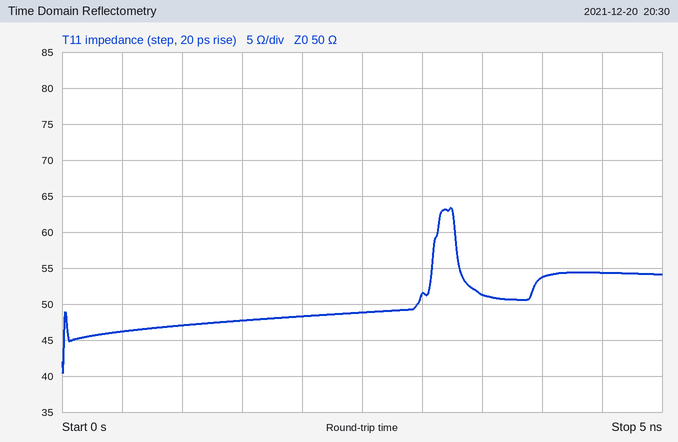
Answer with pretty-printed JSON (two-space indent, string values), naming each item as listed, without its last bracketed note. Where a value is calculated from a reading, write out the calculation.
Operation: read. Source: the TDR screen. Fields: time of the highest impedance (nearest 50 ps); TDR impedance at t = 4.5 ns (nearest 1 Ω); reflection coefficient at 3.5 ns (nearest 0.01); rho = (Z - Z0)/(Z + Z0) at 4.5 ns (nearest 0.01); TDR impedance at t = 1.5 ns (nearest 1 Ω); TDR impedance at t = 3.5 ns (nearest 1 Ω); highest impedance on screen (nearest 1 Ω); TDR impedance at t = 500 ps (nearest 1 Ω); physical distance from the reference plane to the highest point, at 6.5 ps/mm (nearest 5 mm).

{
  "time of the highest impedance": "3.25 ns",
  "TDR impedance at t = 4.5 ns": "54 Ω",
  "reflection coefficient at 3.5 ns": "(51 − 50)/(51 + 50) ≈ +0.01",
  "rho = (Z - Z0)/(Z + Z0) at 4.5 ns": "(54 − 50)/(54 + 50) ≈ +0.04",
  "TDR impedance at t = 1.5 ns": "48 Ω",
  "TDR impedance at t = 3.5 ns": "51 Ω",
  "highest impedance on screen": "63 Ω",
  "TDR impedance at t = 500 ps": "46 Ω",
  "physical distance from the reference plane to the highest point, at 6.5 ps/mm": "3.25 ns / 2 / 6.5 ps/mm ≈ 250 mm"
}
